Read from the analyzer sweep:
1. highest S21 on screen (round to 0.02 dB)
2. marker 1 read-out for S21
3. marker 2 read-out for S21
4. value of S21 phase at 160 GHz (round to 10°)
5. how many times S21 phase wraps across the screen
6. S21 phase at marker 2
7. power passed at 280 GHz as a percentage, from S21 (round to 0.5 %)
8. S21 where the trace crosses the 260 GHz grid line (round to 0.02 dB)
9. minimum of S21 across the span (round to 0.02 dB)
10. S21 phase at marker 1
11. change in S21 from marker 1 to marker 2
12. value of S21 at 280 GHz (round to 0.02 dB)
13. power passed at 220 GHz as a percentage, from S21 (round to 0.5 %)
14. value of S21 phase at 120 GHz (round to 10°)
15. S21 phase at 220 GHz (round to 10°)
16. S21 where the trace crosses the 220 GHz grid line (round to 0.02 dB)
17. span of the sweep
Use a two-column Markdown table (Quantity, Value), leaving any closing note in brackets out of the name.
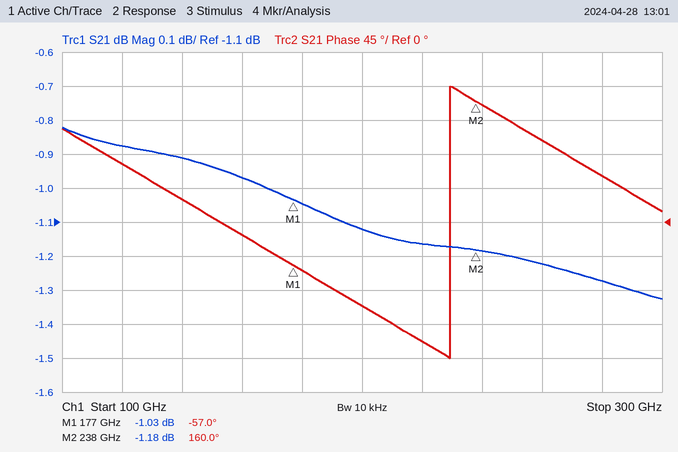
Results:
| Quantity | Value |
|---|---|
| highest S21 on screen | -0.82 dB |
| marker 1 read-out for S21 | -1.03 dB |
| marker 2 read-out for S21 | -1.18 dB |
| value of S21 phase at 160 GHz | -20° |
| how many times S21 phase wraps across the screen | 1 |
| S21 phase at marker 2 | 160.0° |
| power passed at 280 GHz as a percentage, from S21 | 74.5 % |
| S21 where the trace crosses the 260 GHz grid line | -1.22 dB |
| minimum of S21 across the span | -1.32 dB |
| S21 phase at marker 1 | -57.0° |
| change in S21 from marker 1 to marker 2 | -0.15 dB |
| value of S21 at 280 GHz | -1.28 dB |
| power passed at 220 GHz as a percentage, from S21 | 76.5 % |
| value of S21 phase at 120 GHz | 80° |
| S21 phase at 220 GHz | -160° |
| S21 where the trace crosses the 220 GHz grid line | -1.16 dB |
| span of the sweep | 200 GHz |
